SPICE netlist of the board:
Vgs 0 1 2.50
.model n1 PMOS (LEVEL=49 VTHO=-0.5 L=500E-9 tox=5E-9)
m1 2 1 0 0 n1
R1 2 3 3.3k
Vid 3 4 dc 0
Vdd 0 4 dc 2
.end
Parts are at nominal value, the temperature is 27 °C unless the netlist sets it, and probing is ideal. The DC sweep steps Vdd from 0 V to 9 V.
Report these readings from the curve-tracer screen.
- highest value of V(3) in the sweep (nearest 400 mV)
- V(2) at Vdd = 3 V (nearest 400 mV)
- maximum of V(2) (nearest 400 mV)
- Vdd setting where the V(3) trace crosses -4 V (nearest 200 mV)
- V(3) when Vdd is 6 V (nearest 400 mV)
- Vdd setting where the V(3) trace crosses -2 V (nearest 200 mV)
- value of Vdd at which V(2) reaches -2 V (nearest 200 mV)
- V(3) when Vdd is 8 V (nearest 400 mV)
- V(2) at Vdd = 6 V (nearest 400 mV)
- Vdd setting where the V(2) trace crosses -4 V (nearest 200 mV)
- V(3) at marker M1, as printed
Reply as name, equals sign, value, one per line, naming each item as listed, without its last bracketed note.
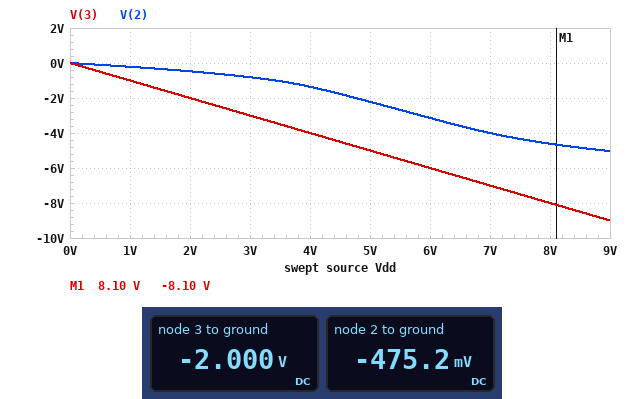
highest value of V(3) in the sweep = 0 V
V(2) at Vdd = 3 V = -800 mV
maximum of V(2) = 0 V
Vdd setting where the V(3) trace crosses -4 V = 4.0 V
V(3) when Vdd is 6 V = -6.0 V
Vdd setting where the V(3) trace crosses -2 V = 2.0 V
value of Vdd at which V(2) reaches -2 V = 4.8 V
V(3) when Vdd is 8 V = -8.0 V
V(2) at Vdd = 6 V = -3.2 V
Vdd setting where the V(2) trace crosses -4 V = 7.0 V
V(3) at marker M1, as printed = -8.10 V
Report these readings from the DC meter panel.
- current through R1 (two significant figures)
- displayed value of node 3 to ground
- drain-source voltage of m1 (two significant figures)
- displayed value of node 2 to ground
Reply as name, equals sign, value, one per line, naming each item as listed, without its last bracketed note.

current through R1 = 460 µA
displayed value of node 3 to ground = -2.000 V
drain-source voltage of m1 = -480 mV
displayed value of node 2 to ground = -475.2 mV
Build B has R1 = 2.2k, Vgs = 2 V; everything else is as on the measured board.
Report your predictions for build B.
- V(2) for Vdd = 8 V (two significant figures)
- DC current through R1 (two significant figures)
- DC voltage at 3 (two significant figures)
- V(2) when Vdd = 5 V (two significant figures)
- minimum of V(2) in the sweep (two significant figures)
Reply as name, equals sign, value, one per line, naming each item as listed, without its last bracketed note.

V(2) for Vdd = 8 V = -5.5 V
DC current through R1 = 490 µA
DC voltage at 3 = -2.0 V
V(2) when Vdd = 5 V = -3.7 V
minimum of V(2) in the sweep = -5.8 V
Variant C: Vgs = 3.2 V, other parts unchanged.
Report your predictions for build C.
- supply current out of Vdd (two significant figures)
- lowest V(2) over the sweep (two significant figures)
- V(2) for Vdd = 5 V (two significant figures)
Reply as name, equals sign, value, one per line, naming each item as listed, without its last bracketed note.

supply current out of Vdd = 490 µA
lowest V(2) over the sweep = -4.4 V
V(2) for Vdd = 5 V = -1.3 V
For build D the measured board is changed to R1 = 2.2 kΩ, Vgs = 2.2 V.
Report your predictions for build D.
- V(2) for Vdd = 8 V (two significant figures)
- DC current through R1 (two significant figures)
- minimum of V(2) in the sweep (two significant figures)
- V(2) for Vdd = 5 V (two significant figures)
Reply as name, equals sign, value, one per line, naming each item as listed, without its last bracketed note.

V(2) for Vdd = 8 V = -5.3 V
DC current through R1 = 550 µA
minimum of V(2) in the sweep = -5.7 V
V(2) for Vdd = 5 V = -3.5 V
